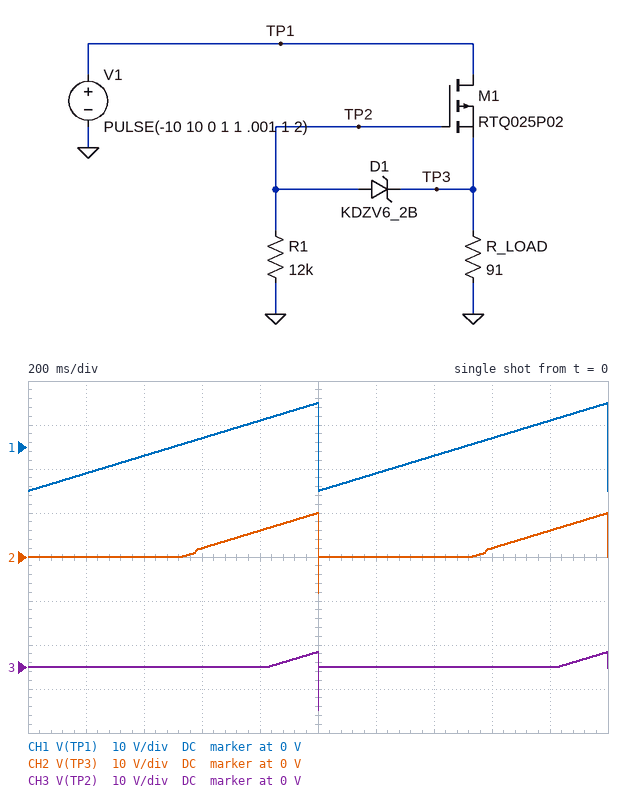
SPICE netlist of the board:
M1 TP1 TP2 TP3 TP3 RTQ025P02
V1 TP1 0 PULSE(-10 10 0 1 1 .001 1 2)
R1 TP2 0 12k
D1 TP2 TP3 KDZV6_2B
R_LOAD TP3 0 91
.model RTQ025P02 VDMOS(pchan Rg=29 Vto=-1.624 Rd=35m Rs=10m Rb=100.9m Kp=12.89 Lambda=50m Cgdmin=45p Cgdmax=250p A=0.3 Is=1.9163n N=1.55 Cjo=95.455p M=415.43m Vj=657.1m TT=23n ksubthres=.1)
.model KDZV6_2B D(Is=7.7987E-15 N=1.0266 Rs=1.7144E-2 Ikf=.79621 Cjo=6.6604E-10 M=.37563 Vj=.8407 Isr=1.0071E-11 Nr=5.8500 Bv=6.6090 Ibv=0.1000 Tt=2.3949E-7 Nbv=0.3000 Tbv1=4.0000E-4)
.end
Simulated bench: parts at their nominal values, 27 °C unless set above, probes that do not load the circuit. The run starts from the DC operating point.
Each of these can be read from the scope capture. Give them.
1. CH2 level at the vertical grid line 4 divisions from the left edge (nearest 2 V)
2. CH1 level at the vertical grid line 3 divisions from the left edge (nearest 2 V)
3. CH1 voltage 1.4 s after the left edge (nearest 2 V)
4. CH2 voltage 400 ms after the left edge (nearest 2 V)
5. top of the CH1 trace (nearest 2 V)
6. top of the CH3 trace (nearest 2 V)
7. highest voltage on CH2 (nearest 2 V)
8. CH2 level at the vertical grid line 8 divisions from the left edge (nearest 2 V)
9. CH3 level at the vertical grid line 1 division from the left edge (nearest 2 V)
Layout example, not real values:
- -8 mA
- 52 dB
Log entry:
- 6 V
- 2 V
- -2 V
- 0 V
- 10 V
- 4 V
- 10 V
- 2 V
- 0 V
